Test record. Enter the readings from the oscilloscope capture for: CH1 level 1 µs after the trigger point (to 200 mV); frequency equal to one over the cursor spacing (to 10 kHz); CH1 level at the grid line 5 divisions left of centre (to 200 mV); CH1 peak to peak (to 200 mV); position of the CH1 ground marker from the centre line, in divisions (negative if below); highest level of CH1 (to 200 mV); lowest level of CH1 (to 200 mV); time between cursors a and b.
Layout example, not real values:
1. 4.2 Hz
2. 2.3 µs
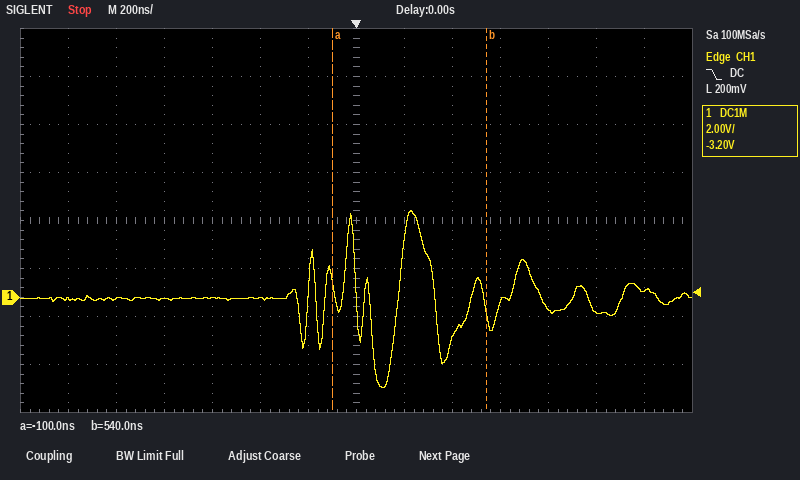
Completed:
1. -600 mV
2. 1.56 MHz
3. 0.0 V
4. 7.4 V
5. -1.6 div
6. 3.6 V
7. -3.8 V
8. 640 ns
